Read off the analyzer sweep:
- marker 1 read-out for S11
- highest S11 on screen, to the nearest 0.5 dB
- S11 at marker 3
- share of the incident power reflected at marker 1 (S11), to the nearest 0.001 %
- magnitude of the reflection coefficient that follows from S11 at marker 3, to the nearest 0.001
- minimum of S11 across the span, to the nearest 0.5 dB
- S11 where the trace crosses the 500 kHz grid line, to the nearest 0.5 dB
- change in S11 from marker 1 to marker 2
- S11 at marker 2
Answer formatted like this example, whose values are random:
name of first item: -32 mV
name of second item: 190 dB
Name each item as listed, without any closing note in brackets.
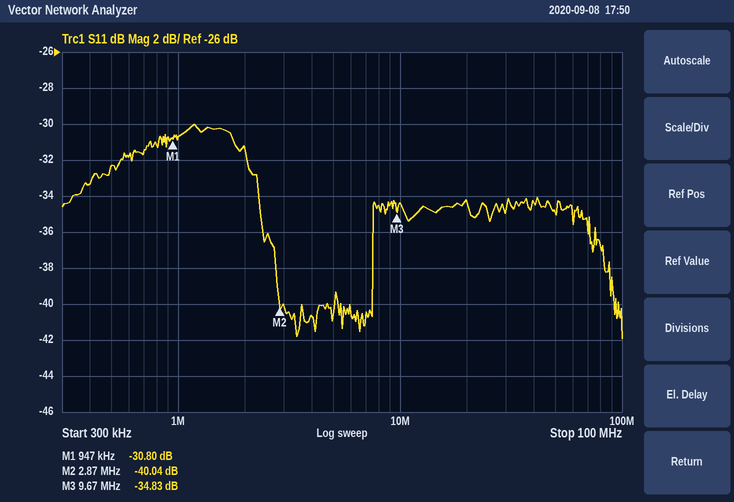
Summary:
marker 1 read-out for S11: -30.80 dB
highest S11 on screen, to the nearest 0.5 dB: -30.0 dB
S11 at marker 3: -34.83 dB
share of the incident power reflected at marker 1 (S11), to the nearest 0.001 %: 0.083 %
magnitude of the reflection coefficient that follows from S11 at marker 3, to the nearest 0.001: 0.018
minimum of S11 across the span, to the nearest 0.5 dB: -42.0 dB
S11 where the trace crosses the 500 kHz grid line, to the nearest 0.5 dB: -32.5 dB
change in S11 from marker 1 to marker 2: -9.24 dB
S11 at marker 2: -40.04 dB
